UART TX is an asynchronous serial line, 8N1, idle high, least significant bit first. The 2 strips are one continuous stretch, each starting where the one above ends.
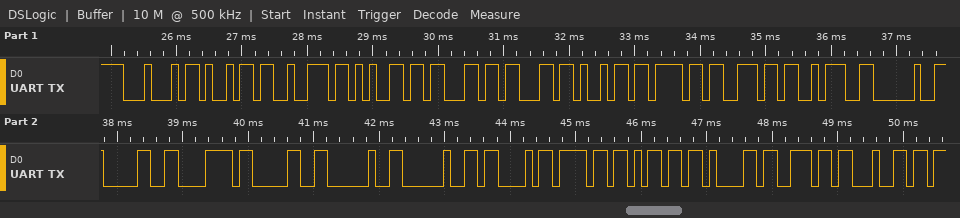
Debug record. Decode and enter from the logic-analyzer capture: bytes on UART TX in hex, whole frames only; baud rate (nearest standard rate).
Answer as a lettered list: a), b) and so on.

a) 44 69 72 65 63 63 69 6F 6E 3A 20 30 78 30 20 20 43 6F 6D 61 6E 64
b) 9600 baud
